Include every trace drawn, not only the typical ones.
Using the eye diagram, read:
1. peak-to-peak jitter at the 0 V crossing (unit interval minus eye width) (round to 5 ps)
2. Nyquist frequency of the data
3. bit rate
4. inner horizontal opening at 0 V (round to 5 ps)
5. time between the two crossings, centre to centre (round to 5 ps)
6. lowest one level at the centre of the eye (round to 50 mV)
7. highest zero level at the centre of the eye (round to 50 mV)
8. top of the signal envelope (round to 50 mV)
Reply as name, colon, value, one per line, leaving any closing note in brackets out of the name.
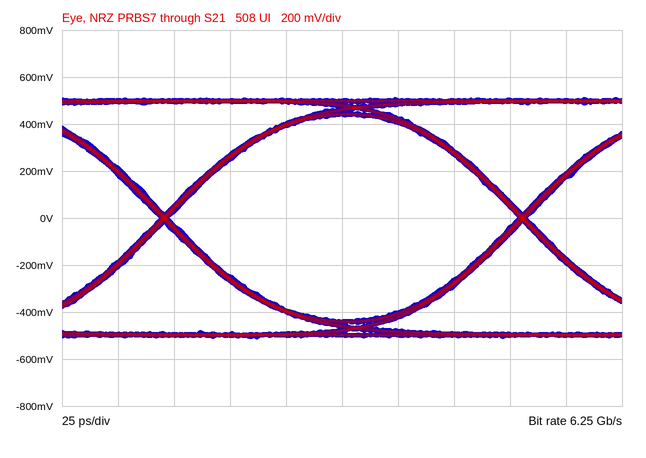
peak-to-peak jitter at the 0 V crossing (unit interval minus eye width): 5 ps
Nyquist frequency of the data: 3.125 GHz
bit rate: 6.25 Gb/s
inner horizontal opening at 0 V: 155 ps
time between the two crossings, centre to centre: 160 ps
lowest one level at the centre of the eye: 450 mV
highest zero level at the centre of the eye: -450 mV
top of the signal envelope: 500 mV
